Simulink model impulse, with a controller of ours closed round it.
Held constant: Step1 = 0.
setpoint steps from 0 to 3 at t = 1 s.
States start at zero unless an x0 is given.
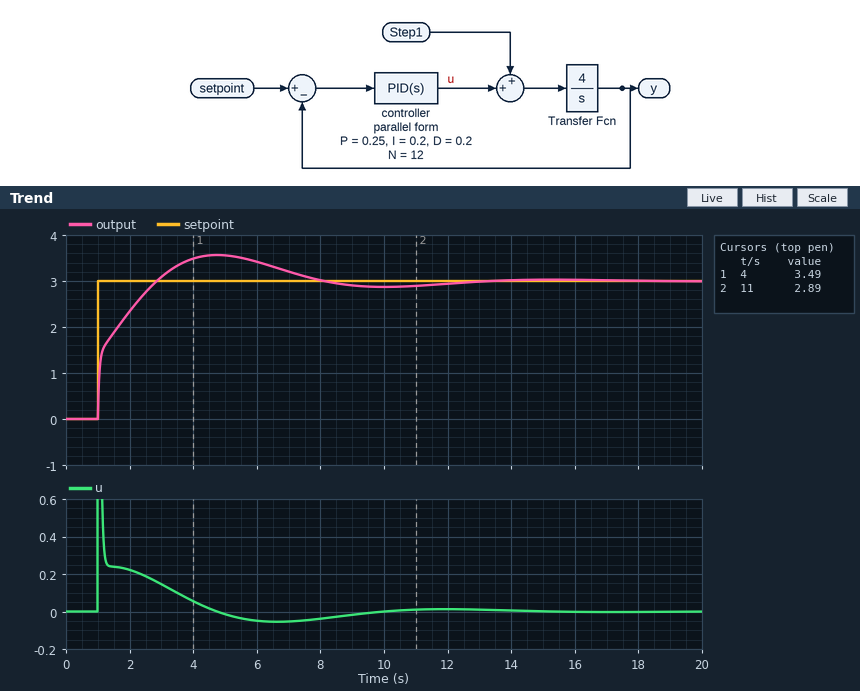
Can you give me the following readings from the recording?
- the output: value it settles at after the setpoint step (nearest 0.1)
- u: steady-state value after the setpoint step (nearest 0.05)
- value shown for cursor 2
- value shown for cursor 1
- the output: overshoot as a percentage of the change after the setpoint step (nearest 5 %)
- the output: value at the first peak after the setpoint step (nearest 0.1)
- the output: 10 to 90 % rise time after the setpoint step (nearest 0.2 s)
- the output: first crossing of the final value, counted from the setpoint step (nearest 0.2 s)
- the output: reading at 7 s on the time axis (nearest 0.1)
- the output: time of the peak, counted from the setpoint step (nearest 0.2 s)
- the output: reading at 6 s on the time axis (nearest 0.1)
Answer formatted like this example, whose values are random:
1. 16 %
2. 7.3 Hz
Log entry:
1. 3.0
2. 0.00
3. 2.89
4. 3.49
5. 20 %
6. 3.6
7. 1.4 s
8. 1.8 s
9. 3.2
10. 3.8 s
11. 3.4
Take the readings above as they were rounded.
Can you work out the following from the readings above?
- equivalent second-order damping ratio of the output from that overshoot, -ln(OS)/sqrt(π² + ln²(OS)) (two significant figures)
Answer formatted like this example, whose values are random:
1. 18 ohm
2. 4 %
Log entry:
1. 0.46
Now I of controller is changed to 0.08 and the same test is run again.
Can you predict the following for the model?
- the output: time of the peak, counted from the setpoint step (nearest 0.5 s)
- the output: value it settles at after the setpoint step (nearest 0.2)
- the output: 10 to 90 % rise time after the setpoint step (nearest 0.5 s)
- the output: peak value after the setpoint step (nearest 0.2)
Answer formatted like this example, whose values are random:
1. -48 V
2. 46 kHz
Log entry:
1. 5.5 s
2. 3.0
3. 2.0 s
4. 3.4
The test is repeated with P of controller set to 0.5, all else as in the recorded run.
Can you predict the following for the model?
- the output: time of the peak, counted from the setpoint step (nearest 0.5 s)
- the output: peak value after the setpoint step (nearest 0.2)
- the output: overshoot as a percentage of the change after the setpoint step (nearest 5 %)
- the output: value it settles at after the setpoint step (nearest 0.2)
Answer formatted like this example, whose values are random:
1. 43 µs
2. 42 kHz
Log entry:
1. 3.0 s
2. 3.2
3. 10 %
4. 3.0
